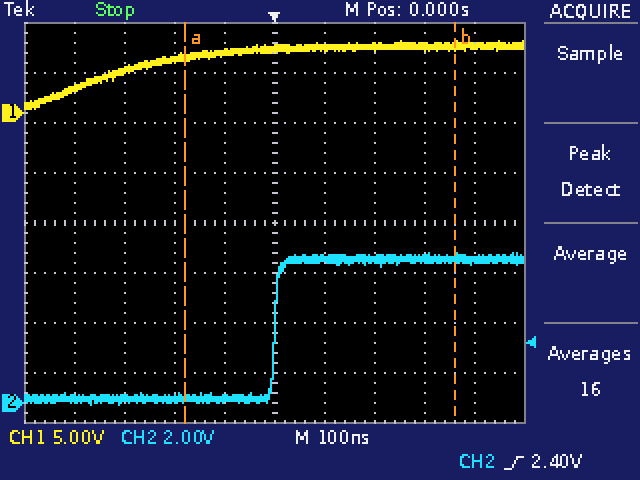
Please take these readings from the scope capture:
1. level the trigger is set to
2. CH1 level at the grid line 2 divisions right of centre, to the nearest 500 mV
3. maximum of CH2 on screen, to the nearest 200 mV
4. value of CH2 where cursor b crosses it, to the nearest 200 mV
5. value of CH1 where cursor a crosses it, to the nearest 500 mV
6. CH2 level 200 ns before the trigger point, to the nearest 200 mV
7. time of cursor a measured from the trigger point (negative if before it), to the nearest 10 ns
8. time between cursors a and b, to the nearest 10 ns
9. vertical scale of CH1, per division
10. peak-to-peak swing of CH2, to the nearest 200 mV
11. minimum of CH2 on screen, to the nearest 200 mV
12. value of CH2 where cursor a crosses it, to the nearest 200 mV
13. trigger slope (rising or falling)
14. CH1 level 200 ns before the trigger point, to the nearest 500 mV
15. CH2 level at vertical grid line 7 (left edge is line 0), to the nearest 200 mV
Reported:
2.40 V
6.5 V
6.0 V
5.8 V
5.5 V
200 mV
-180 ns
540 ns
5 V
6.0 V
0.0 V
200 mV
rising
5.5 V
5.8 V
